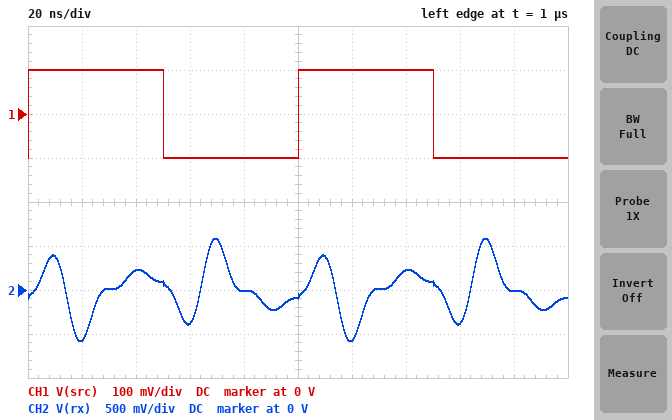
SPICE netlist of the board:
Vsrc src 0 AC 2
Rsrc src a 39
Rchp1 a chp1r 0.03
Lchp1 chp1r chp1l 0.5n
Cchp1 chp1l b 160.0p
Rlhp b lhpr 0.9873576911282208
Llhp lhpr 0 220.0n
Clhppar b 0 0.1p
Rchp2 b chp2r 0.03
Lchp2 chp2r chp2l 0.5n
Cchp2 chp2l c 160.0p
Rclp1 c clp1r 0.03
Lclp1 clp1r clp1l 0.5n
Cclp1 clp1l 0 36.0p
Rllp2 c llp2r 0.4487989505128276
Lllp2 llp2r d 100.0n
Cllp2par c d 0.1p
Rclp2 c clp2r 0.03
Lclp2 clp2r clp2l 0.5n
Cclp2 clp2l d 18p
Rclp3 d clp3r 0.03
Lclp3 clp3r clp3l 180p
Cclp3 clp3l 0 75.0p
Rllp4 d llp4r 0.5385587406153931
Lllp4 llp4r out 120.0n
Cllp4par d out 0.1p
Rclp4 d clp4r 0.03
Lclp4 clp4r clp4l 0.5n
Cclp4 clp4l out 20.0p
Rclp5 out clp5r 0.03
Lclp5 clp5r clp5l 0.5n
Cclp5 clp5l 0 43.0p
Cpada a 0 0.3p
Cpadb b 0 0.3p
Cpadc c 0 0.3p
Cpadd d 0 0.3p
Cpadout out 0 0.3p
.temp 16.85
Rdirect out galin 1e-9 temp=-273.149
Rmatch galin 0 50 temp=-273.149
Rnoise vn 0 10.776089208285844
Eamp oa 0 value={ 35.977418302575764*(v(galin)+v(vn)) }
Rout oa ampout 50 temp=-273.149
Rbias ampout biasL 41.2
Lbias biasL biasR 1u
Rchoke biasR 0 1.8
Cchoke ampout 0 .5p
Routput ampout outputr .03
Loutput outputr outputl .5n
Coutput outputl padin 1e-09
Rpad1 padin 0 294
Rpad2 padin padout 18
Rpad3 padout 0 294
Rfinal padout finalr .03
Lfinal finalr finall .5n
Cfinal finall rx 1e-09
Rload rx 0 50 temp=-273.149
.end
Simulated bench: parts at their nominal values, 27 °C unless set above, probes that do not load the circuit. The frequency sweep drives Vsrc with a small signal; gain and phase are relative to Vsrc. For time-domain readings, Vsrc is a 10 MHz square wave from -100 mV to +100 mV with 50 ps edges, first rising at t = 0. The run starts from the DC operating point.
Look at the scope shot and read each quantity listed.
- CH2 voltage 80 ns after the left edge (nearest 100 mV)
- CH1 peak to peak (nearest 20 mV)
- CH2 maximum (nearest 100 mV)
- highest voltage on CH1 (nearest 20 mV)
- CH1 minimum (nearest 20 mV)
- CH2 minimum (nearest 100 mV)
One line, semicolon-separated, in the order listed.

0 V; 200 mV; 600 mV; 100 mV; -100 mV; -600 mV
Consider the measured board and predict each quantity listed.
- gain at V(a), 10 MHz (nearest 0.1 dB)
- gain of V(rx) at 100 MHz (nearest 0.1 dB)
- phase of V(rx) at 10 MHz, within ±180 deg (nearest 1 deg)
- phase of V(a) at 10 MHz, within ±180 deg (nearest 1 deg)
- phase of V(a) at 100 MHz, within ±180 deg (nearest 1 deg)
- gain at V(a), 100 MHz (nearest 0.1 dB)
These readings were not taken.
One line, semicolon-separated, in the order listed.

-0.9 dB; -35.0 dB; -140 deg; -25 deg; -17 deg; -0.4 dB
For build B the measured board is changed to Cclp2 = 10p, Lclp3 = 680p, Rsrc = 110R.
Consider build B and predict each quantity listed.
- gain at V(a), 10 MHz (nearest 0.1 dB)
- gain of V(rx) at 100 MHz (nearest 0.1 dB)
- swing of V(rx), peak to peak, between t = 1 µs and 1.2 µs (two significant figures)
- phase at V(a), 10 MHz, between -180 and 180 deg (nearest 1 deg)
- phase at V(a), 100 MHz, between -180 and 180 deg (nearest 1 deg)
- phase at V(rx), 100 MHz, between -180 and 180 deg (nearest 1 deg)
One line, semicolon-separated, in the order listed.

-4.4 dB; -26.8 dB; 650 mV; -52 deg; -18 deg; 33 deg
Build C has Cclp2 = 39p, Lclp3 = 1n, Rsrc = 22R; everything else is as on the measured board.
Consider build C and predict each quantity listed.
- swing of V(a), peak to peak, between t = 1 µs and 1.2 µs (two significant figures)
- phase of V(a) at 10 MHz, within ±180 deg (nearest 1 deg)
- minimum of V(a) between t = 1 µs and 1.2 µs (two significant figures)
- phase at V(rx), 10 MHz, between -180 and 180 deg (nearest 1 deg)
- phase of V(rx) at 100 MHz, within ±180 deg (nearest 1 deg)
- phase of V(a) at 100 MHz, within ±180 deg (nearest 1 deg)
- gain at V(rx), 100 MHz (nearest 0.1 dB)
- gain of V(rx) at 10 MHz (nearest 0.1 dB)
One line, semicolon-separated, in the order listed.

230 mV; -15 deg; -110 mV; -130 deg; -148 deg; -18 deg; -33.2 dB; -2.6 dB
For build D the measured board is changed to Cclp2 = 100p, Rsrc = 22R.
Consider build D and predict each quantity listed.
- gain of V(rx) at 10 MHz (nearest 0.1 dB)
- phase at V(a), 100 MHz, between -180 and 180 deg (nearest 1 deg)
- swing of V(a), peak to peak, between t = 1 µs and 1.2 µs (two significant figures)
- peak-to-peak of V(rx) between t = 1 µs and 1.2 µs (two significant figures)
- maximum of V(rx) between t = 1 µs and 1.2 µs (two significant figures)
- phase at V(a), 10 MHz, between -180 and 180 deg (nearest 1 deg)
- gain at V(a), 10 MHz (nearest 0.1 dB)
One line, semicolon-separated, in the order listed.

-2.6 dB; -24 deg; 220 mV; 820 mV; 410 mV; -15 deg; -0.3 dB
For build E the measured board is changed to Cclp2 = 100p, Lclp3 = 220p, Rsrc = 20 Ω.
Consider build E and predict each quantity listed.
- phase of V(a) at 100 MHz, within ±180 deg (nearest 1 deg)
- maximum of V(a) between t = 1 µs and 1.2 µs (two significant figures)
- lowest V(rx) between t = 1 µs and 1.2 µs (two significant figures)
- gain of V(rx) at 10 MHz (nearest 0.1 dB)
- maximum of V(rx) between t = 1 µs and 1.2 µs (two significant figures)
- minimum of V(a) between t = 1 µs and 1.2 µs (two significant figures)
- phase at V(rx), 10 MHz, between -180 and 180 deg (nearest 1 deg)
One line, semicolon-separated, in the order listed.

-22 deg; 110 mV; -420 mV; -2.6 dB; 420 mV; -110 mV; -129 deg
